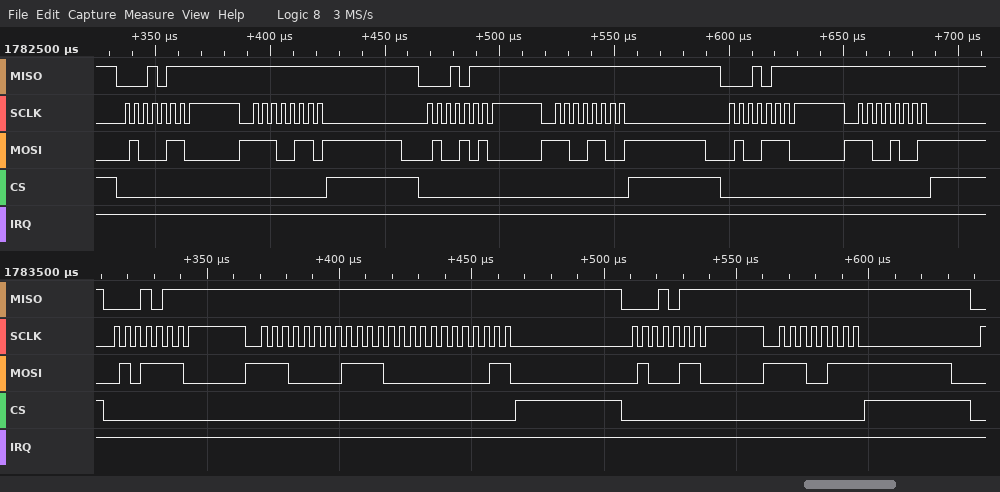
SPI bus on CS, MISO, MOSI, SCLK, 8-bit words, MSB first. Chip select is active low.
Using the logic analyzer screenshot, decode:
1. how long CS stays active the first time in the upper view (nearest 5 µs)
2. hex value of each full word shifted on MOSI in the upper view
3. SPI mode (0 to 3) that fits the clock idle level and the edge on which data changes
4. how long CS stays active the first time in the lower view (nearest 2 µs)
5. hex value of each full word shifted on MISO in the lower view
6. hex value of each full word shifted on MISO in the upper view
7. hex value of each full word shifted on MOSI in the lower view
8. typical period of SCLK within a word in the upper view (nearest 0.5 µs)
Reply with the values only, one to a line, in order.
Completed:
90 µs
46, E6, 4A, CC, 4E, C9
0
156 µs
17, FF, FF, FF, 17, FF
17, FF, 17, FF, 17, FF
5E, E0, F0, 03, 46, E7
4 µs
